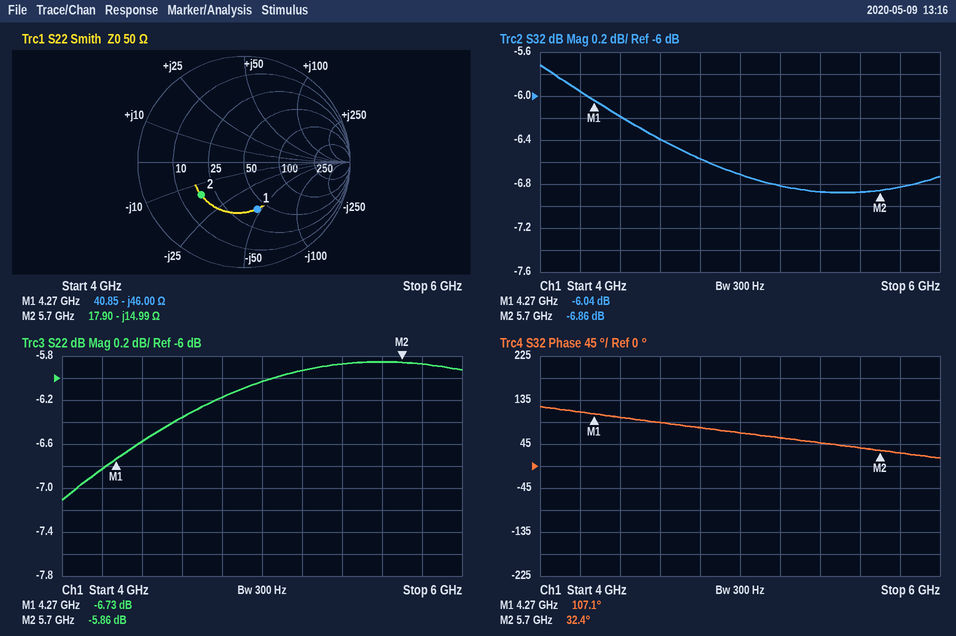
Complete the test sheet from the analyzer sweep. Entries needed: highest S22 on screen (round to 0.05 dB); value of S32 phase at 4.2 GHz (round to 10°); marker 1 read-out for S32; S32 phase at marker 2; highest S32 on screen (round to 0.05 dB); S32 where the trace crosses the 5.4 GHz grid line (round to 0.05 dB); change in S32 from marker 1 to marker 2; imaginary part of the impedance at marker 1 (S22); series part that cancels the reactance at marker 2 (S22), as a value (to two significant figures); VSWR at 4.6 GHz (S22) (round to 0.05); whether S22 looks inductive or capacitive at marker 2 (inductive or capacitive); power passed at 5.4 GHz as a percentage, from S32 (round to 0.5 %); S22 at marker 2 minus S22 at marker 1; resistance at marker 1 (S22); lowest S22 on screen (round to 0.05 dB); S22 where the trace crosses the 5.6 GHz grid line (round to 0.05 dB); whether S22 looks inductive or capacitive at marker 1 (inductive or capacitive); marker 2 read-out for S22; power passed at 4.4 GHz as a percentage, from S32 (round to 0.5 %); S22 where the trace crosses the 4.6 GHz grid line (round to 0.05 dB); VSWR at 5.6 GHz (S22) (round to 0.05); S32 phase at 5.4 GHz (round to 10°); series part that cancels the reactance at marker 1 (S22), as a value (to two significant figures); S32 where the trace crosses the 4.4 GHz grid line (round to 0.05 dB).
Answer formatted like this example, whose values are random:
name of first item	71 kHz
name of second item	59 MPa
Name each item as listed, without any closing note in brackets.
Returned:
highest S22 on screen	-5.85 dB
value of S32 phase at 4.2 GHz	110°
marker 1 read-out for S32	-6.04 dB
S32 phase at marker 2	32.4°
highest S32 on screen	-5.70 dB
S32 where the trace crosses the 5.4 GHz grid line	-6.85 dB
change in S32 from marker 1 to marker 2	-0.82 dB
imaginary part of the impedance at marker 1	-46.00 Ω
series part that cancels the reactance at marker 2 (S22), as a value	420 pH
VSWR at 4.6 GHz (S22)	2.85
whether S22 looks inductive or capacitive at marker 2	capacitive
power passed at 5.4 GHz as a percentage, from S32	20.5 %
S22 at marker 2 minus S22 at marker 1	0.87 dB
resistance at marker 1	40.85 Ω
lowest S22 on screen	-7.10 dB
S22 where the trace crosses the 5.6 GHz grid line	-5.85 dB
whether S22 looks inductive or capacitive at marker 1	capacitive
marker 2 read-out for S22	-5.86 dB
power passed at 4.4 GHz as a percentage, from S32	24.0 %
S22 where the trace crosses the 4.6 GHz grid line	-6.35 dB
VSWR at 5.6 GHz (S22)	3.10
S32 phase at 5.4 GHz	50°
series part that cancels the reactance at marker 1 (S22), as a value	1.7 nH
S32 where the trace crosses the 4.4 GHz grid line	-6.20 dB
